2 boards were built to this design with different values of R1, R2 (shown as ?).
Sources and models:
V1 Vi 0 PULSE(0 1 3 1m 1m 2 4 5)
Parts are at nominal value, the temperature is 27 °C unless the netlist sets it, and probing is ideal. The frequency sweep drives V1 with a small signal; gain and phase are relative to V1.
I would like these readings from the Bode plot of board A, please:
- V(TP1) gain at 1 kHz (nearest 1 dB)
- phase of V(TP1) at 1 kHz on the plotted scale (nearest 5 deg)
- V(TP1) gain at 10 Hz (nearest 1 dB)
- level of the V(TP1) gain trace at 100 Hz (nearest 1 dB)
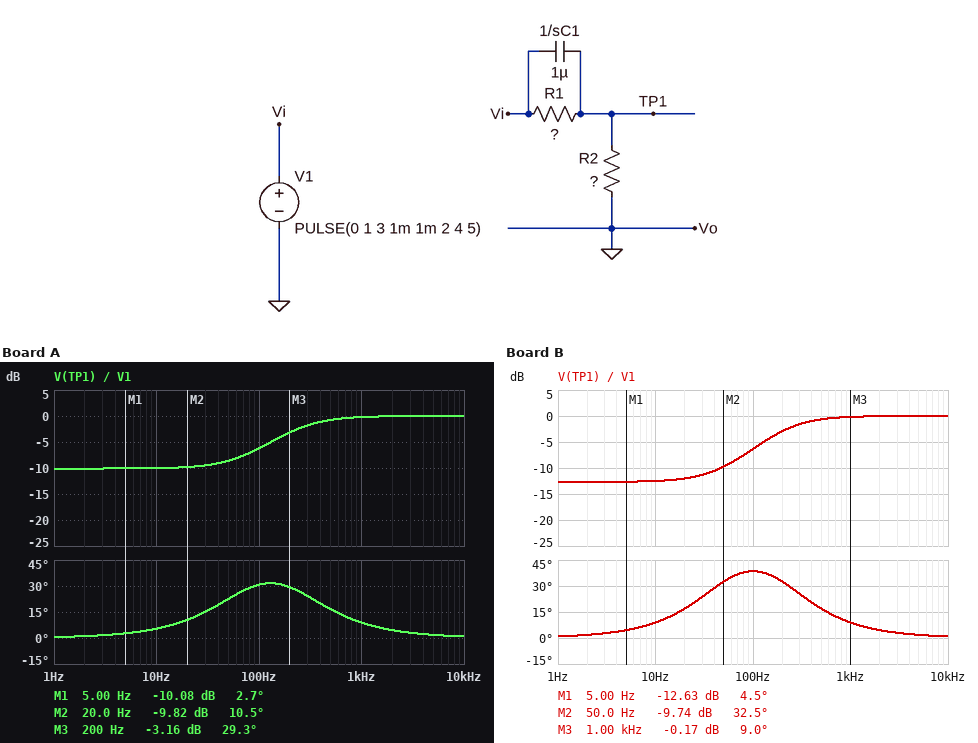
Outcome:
0 dB
10 deg
-10 dB
-6 dB
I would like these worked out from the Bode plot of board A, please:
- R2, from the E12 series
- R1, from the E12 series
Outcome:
1 kΩ
2.2 kΩ
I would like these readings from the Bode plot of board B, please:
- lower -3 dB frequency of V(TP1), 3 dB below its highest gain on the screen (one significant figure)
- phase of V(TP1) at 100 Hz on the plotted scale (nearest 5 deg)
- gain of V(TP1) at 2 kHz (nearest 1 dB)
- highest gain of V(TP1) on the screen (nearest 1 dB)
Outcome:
200 Hz
40 deg
0 dB
0 dB
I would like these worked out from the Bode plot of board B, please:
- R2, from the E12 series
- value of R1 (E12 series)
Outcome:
1 kΩ
3.3 kΩ
